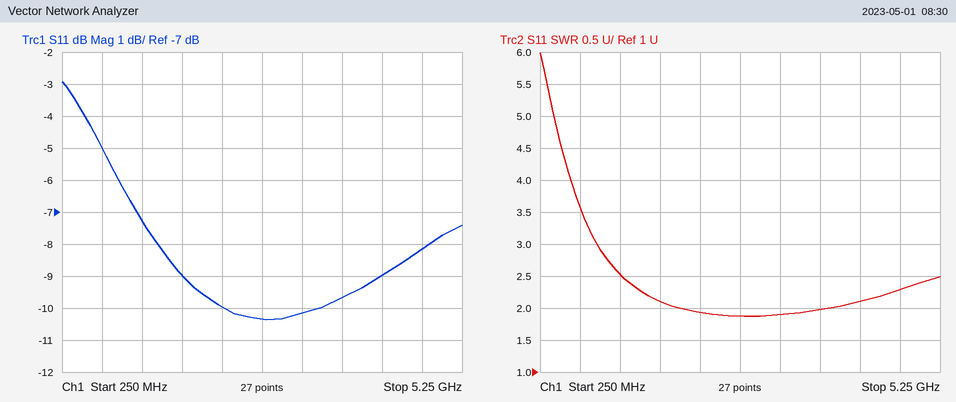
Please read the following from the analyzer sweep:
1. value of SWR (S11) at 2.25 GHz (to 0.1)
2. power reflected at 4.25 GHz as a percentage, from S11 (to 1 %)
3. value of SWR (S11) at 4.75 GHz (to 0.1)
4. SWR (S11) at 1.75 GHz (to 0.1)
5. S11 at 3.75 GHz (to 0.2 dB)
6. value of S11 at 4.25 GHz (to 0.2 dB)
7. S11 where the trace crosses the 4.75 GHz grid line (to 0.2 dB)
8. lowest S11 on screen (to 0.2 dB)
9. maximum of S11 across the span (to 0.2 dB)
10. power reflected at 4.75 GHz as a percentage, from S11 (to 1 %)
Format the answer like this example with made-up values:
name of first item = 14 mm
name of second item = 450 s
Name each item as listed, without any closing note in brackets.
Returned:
value of SWR (S11) at 2.25 GHz = 1.9
power reflected at 4.25 GHz as a percentage, from S11 = 13 %
value of SWR (S11) at 4.75 GHz = 2.3
SWR (S11) at 1.75 GHz = 2.1
S11 at 3.75 GHz = -9.6 dB
value of S11 at 4.25 GHz = -9.0 dB
S11 where the trace crosses the 4.75 GHz grid line = -8.2 dB
lowest S11 on screen = -10.4 dB
maximum of S11 across the span = -3.0 dB
power reflected at 4.75 GHz as a percentage, from S11 = 15 %
